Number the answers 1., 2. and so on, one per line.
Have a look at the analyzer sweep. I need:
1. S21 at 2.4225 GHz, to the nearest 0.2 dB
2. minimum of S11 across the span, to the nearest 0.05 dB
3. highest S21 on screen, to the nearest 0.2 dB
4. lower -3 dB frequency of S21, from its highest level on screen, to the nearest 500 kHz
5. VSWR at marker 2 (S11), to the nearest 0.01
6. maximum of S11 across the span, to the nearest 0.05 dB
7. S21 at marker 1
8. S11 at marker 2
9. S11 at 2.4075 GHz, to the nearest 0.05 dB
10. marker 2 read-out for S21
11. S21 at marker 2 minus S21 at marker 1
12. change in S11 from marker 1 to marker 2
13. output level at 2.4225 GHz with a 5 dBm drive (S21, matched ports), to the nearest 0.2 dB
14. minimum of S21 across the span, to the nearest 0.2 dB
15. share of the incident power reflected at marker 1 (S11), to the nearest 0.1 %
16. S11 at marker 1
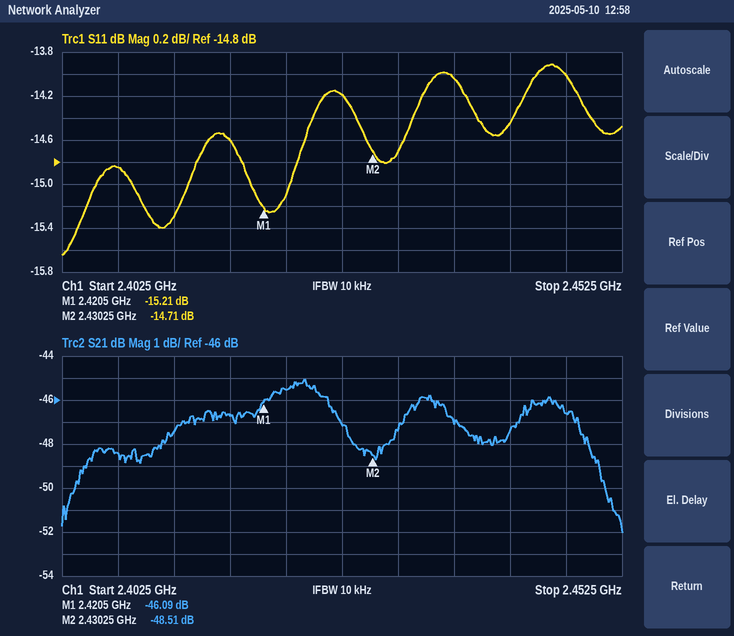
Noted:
1. -45.6 dB
2. -15.65 dB
3. -45.0 dB
4. 2.4115 GHz
5. 1.45
6. -13.90 dB
7. -46.09 dB
8. -14.71 dB
9. -14.85 dB
10. -48.51 dB
11. -2.42 dB
12. 0.50 dB
13. -40.6 dBm
14. -52.0 dB
15. 3.0 %
16. -15.21 dB
